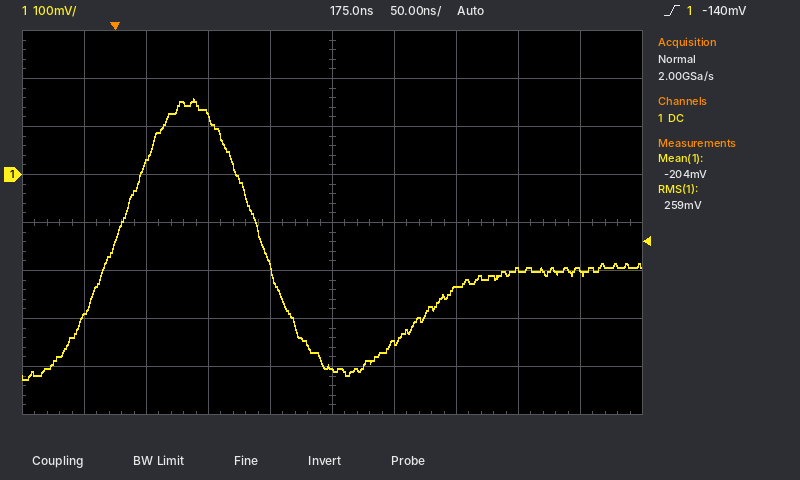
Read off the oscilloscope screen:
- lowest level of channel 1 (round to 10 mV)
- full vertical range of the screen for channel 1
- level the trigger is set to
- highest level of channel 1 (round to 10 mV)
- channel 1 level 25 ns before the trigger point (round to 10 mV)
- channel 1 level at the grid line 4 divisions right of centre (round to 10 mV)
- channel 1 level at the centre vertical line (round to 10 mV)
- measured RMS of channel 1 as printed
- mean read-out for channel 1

-430 mV
800 mV
-140 mV
160 mV
-290 mV
-200 mV
-410 mV
259 mV
-204 mV
